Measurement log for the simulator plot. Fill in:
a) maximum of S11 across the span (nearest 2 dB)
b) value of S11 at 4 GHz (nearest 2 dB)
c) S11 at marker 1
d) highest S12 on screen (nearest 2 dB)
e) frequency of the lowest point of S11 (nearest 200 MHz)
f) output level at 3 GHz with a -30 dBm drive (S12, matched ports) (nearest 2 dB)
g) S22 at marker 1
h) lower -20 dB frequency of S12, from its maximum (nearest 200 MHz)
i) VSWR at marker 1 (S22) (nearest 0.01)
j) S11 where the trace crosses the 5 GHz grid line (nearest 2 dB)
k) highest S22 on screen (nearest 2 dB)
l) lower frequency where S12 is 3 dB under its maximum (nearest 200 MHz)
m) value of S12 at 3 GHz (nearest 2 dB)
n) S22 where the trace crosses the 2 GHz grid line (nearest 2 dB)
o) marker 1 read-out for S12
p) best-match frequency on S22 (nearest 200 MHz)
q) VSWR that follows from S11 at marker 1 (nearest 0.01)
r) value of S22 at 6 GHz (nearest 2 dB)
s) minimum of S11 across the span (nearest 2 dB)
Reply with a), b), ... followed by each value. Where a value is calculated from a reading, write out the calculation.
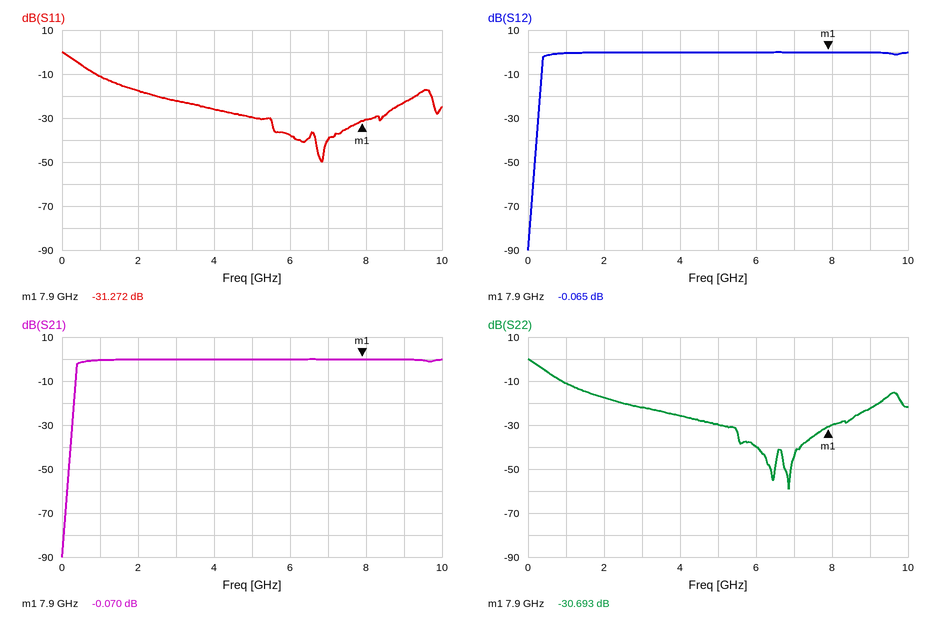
a) 0 dB
b) -26 dB
c) -31.272 dB
d) 0 dB
e) 6.8 GHz
f) -30 dBm + (0 dB) = -30 dBm
g) -30.693 dB
h) 400 MHz
i) (1 + 0.0292)/(1 − 0.0292) ≈ 1.06
j) -30 dB
k) 0 dB
l) 400 MHz
m) 0 dB
n) -18 dB
o) -0.065 dB
p) 6.8 GHz
q) (1 + 0.0273)/(1 − 0.0273) ≈ 1.06
r) -40 dB
s) -50 dB
